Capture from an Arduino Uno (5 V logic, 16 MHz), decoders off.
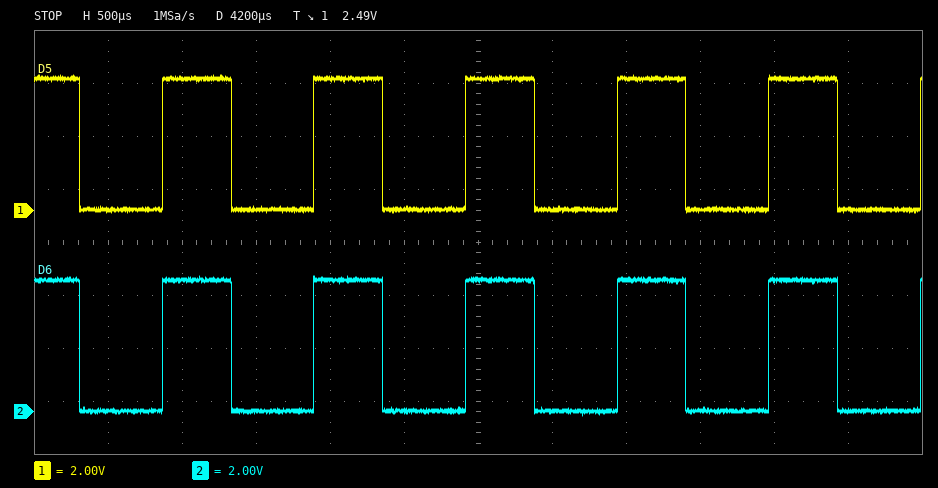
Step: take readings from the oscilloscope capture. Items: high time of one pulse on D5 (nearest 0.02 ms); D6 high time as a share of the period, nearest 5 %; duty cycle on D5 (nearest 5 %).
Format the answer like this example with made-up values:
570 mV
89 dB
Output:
0.46 ms
45 %
45 %
